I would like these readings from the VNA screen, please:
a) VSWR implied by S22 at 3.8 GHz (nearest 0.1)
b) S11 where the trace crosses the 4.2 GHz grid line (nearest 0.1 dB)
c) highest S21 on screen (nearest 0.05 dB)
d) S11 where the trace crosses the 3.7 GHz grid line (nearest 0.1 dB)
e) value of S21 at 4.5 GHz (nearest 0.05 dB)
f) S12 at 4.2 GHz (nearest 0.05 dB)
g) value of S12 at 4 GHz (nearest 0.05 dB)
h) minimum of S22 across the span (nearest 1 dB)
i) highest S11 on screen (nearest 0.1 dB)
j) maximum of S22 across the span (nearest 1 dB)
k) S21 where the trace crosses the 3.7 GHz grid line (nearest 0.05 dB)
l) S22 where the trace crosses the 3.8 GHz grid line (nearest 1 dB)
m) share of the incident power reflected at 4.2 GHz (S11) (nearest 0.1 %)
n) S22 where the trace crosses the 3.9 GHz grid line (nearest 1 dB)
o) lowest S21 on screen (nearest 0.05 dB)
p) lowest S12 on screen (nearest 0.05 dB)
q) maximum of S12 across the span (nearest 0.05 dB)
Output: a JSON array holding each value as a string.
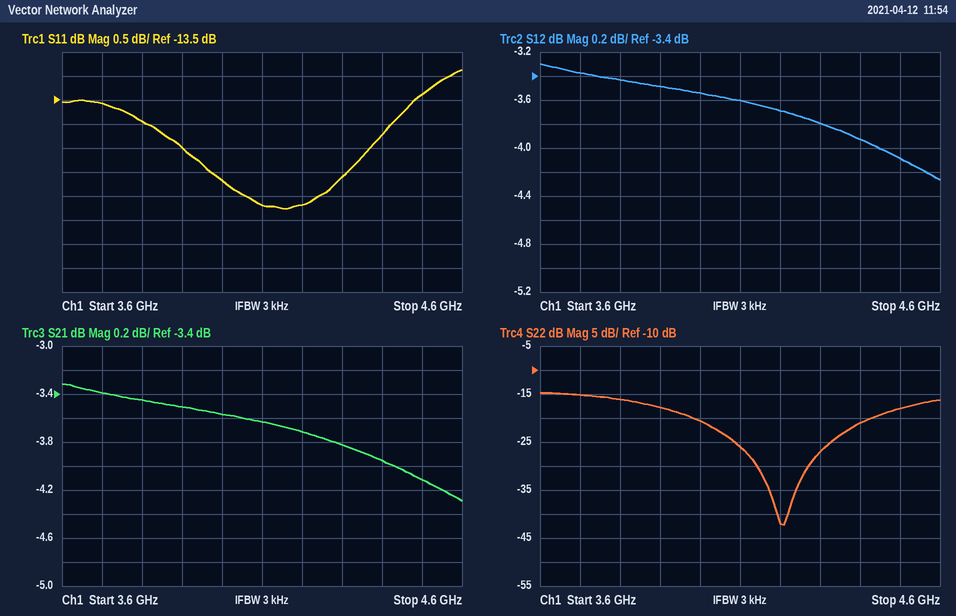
["1.4", "-15.7 dB", "-3.30 dB", "-13.6 dB", "-4.10 dB", "-3.70 dB", "-3.55 dB", "-42 dB", "-12.9 dB", "-15 dB", "-3.40 dB", "-16 dB", "2.7 %", "-18 dB", "-4.30 dB", "-4.25 dB", "-3.30 dB"]
